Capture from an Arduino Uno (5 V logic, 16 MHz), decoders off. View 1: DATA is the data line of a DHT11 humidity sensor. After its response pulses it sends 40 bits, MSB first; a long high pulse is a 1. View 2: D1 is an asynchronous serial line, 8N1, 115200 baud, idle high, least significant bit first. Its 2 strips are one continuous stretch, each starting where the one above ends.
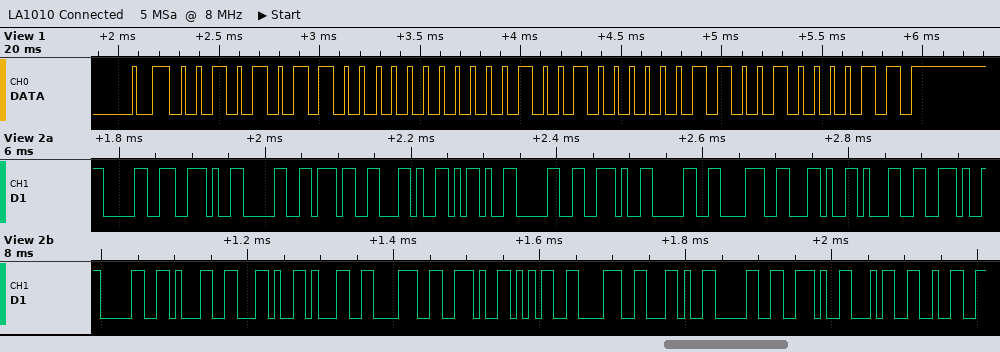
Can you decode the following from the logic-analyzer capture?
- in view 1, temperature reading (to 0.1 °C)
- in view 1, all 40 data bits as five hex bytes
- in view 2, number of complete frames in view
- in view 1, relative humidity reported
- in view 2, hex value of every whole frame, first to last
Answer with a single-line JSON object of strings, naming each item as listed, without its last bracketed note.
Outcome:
{"in view 1, temperature reading": "18.6 °C", "in view 1, all 40 data bits as five hex bytes": "2B 00 12 06 43", "in view 2, number of complete frames in view": "26", "in view 1, relative humidity reported": "43 %", "in view 2, hex value of every whole frame, first to last": "30 2E 30 37 2C 2D 30 2E 30 38 2C 31 2E 30 31 2C 31 38 2E 35 38 2C 30 2E 34 32"}
